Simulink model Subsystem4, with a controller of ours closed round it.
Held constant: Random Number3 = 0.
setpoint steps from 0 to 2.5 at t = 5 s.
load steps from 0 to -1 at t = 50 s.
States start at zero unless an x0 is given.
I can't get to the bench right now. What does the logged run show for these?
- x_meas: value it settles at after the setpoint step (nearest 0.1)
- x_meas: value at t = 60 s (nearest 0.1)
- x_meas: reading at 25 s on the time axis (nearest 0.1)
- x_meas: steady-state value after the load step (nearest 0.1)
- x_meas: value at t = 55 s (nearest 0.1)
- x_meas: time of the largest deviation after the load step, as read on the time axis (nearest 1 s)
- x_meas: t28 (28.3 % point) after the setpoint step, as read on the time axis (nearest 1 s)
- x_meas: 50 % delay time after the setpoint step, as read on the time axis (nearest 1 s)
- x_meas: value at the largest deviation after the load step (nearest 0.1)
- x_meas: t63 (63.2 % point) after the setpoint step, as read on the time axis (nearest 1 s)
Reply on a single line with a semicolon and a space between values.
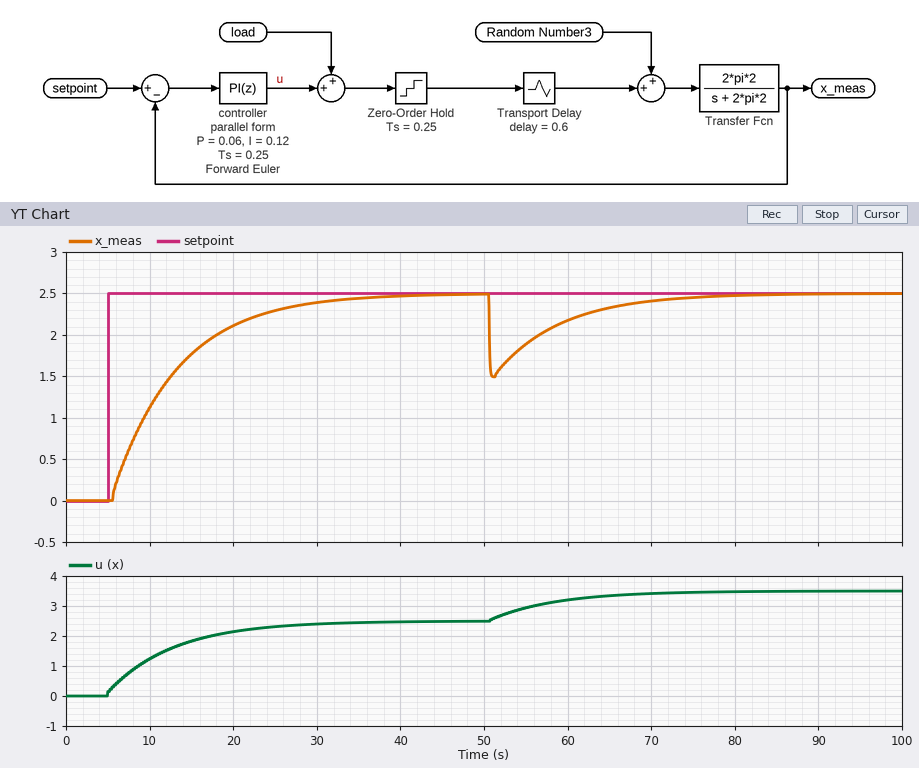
2.5; 2.2; 2.3; 2.5; 1.9; 51 s; 8 s; 11 s; 1.5; 13 s
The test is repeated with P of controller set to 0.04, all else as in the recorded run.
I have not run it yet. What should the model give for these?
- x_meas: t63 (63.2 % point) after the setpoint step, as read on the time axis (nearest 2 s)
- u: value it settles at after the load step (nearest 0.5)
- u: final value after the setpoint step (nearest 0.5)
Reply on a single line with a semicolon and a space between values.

14 s; 3.5; 2.5
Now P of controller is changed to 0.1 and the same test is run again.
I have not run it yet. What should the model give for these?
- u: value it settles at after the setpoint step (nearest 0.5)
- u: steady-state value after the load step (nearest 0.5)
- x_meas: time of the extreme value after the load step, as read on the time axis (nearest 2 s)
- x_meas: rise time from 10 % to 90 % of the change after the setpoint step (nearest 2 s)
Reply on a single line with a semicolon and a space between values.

2.5; 3.5; 52 s; 18 s
